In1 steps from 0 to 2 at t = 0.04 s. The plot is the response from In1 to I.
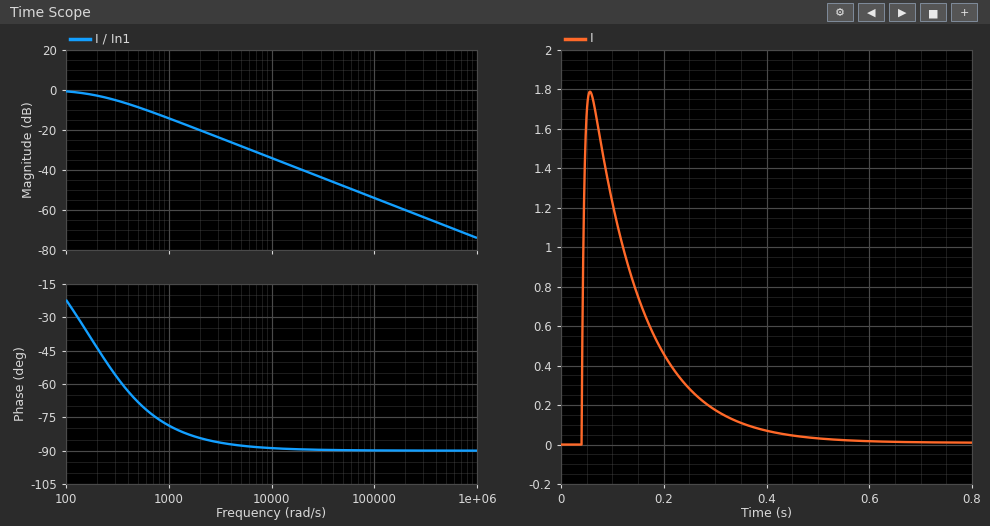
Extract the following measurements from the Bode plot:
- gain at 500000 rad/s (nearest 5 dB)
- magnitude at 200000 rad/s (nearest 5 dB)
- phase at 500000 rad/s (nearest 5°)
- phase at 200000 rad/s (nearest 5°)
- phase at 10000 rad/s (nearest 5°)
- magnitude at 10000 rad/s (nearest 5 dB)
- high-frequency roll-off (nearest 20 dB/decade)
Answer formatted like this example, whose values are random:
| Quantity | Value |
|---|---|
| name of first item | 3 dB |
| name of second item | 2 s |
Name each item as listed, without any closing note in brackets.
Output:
| Quantity | Value |
|---|---|
| gain at 500000 rad/s | -70 dB |
| magnitude at 200000 rad/s | -60 dB |
| phase at 500000 rad/s | -90° |
| phase at 200000 rad/s | -90° |
| phase at 10000 rad/s | -90° |
| magnitude at 10000 rad/s | -35 dB |
| high-frequency roll-off | -20 dB/decade |
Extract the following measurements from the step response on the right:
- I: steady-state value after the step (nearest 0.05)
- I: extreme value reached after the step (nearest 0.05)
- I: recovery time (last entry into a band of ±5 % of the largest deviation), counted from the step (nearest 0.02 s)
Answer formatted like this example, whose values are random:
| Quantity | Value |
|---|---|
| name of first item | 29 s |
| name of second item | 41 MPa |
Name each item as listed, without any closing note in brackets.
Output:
| Quantity | Value |
|---|---|
| I: steady-state value after the step | 0.00 |
| I: extreme value reached after the step | 1.80 |
| I: recovery time (last entry into a band of ±5 % of the largest deviation), counted from the step | 0.32 s |
